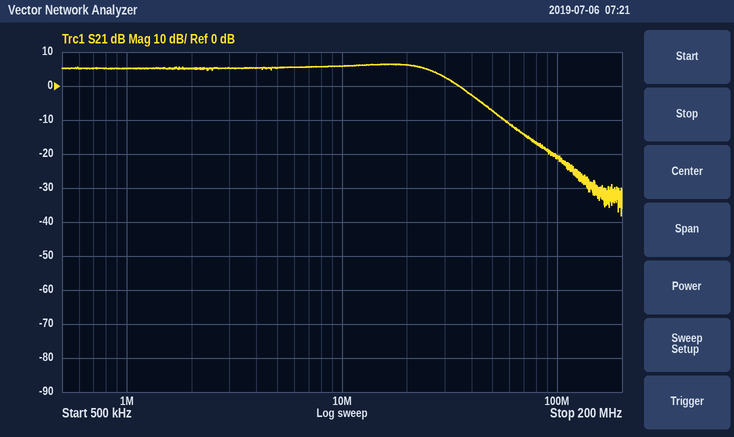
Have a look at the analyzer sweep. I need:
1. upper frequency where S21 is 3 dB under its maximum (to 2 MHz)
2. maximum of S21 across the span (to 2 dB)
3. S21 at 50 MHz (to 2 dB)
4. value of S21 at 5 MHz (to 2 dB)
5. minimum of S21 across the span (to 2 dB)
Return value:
28 MHz
6 dB
-8 dB
6 dB
-38 dB
